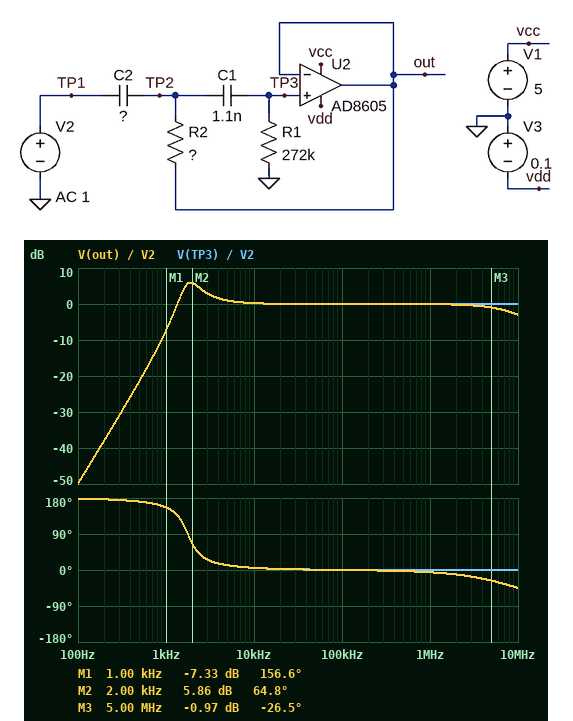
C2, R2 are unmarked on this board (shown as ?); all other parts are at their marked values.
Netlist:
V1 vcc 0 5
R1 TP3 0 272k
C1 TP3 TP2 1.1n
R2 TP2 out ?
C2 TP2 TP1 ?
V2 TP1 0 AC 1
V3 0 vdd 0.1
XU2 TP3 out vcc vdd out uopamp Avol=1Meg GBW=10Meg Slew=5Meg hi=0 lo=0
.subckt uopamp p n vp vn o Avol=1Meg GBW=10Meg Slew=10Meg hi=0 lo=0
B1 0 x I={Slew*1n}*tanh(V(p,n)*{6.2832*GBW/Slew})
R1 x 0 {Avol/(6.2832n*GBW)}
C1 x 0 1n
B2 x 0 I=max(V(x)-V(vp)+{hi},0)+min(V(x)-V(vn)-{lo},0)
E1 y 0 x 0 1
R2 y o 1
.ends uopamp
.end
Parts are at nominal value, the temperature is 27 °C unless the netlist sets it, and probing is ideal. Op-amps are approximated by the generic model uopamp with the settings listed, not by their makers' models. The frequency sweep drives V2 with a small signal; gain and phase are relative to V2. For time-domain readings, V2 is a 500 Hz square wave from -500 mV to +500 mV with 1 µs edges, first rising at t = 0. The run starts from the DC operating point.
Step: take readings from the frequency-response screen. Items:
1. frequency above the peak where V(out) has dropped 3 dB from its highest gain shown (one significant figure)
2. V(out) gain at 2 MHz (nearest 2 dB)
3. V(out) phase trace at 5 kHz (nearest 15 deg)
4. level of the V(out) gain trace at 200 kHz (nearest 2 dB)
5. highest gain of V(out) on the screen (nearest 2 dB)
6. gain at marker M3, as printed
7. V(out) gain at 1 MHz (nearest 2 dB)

3 kHz
0 dB
15 deg
0 dB
6 dB
-0.97 dB
0 dB
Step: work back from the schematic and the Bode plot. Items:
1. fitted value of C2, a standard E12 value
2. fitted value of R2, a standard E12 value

1.5 nF
18 kΩ
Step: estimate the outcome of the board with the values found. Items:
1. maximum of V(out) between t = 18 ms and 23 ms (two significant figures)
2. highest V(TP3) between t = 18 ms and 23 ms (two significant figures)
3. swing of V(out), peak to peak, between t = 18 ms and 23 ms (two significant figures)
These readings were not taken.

990 mV
990 mV
1.1 V
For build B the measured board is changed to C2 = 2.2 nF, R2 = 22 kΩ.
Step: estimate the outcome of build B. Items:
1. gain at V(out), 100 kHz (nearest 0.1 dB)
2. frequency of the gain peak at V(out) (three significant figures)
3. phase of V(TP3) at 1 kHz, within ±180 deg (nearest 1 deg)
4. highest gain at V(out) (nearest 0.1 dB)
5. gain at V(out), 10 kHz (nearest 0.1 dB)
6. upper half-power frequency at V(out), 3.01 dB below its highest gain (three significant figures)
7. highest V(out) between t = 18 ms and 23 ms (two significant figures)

0 dB
1.46 kHz
133 deg
4.8 dB
0.1 dB
2.68 kHz
1.0 V
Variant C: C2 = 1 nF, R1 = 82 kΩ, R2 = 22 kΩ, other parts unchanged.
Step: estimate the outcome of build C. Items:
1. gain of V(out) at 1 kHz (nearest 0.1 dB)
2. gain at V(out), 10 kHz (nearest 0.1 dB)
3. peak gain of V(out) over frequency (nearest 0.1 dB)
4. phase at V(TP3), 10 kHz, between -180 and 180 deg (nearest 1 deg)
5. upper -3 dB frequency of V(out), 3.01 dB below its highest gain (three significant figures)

-21.8 dB
0.5 dB
1.0 dB
23 deg
7.57 MHz
